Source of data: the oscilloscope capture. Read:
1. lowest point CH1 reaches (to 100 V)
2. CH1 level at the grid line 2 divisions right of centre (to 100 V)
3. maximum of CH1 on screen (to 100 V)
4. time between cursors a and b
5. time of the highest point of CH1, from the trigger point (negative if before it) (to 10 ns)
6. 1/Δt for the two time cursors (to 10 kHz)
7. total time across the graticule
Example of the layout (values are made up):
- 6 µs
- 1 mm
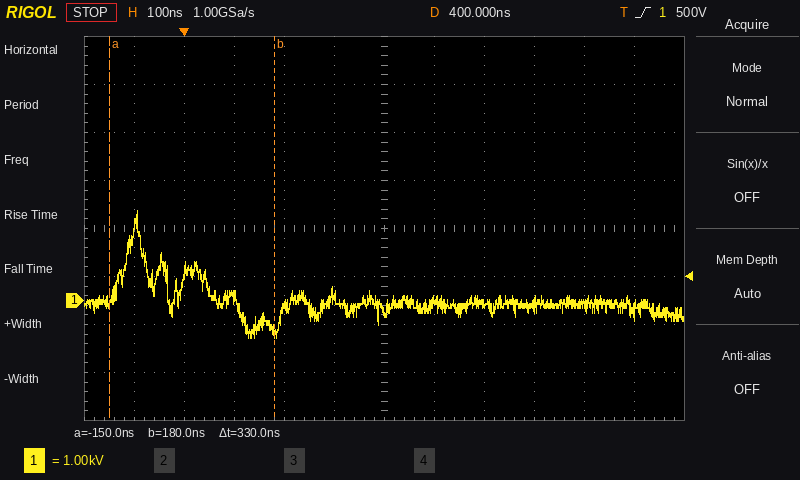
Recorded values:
- -800 V
- -100 V
- 1.9 kV
- 330 ns
- -90 ns
- 3.03 MHz
- 1.2 µs
